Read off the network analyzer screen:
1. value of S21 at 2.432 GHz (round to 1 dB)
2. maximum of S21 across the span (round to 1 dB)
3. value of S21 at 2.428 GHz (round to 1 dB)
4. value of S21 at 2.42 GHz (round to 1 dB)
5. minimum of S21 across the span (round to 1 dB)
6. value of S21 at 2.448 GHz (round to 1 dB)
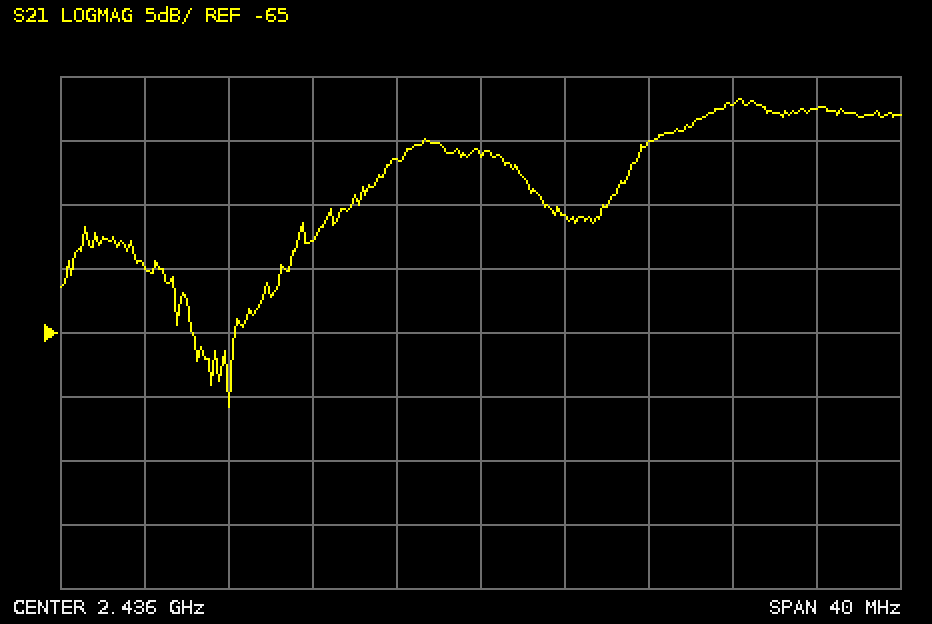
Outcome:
-51 dB
-47 dB
-58 dB
-60 dB
-71 dB
-47 dB
